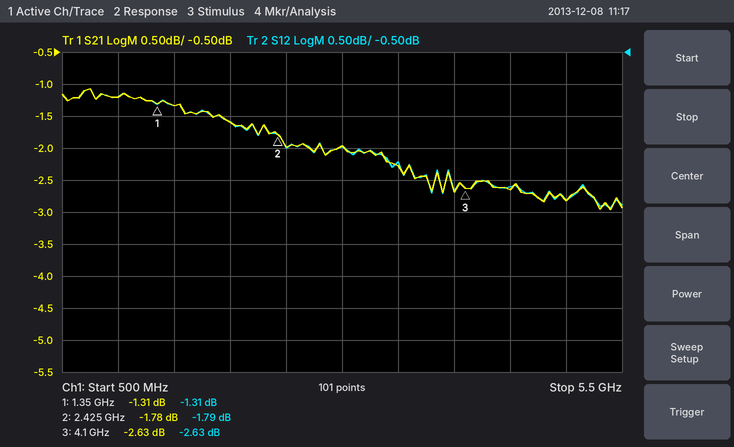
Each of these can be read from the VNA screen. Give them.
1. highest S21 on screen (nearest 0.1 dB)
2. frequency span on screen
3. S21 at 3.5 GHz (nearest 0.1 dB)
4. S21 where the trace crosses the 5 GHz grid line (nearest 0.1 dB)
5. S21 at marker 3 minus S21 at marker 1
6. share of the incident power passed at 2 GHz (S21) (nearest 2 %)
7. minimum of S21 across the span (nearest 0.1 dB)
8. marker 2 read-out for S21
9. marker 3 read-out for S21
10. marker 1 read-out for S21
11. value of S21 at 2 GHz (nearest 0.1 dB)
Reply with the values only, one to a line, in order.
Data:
-1.1 dB
5 GHz
-2.3 dB
-2.8 dB
-1.32 dB
70 %
-3.0 dB
-1.78 dB
-2.63 dB
-1.31 dB
-1.6 dB
